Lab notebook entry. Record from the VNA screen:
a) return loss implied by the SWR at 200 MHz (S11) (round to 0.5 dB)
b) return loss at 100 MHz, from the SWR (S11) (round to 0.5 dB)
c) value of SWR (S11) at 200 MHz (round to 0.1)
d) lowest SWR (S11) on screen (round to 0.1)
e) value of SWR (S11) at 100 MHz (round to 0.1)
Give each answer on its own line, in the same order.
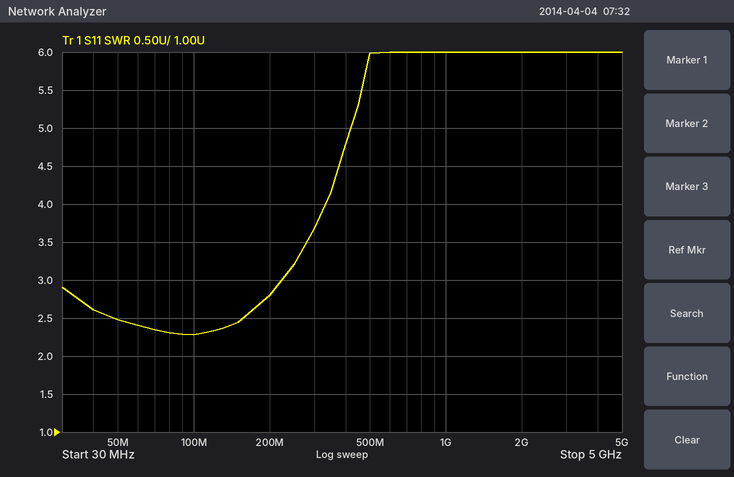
6.5 dB
8.0 dB
2.8
2.3
2.3
